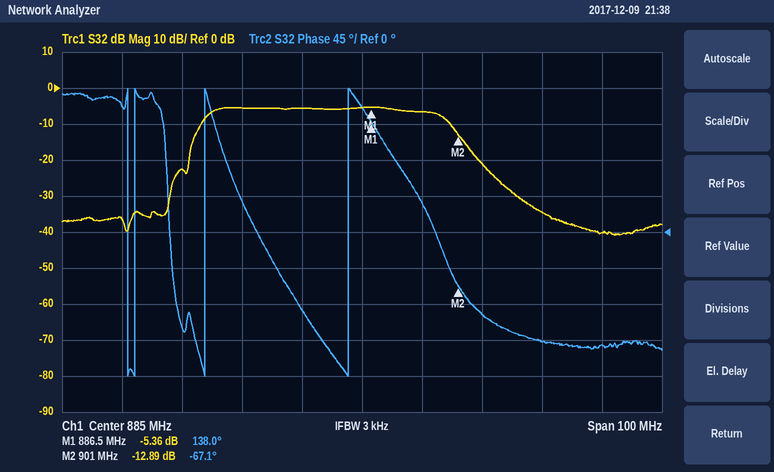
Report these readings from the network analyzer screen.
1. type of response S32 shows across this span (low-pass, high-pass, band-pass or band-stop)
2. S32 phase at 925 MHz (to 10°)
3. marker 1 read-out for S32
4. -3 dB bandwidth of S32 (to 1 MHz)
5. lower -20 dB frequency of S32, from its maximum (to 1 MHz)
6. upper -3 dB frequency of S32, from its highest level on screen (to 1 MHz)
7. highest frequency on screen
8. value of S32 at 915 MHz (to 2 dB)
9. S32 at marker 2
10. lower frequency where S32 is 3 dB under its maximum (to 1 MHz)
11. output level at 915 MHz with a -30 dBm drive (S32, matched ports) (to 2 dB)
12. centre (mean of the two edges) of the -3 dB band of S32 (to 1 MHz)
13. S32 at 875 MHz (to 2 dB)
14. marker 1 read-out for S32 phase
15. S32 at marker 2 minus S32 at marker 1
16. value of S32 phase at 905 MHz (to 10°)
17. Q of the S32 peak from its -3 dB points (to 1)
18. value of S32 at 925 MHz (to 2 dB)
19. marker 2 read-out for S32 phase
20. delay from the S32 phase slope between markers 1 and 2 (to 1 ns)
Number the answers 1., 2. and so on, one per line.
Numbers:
1. band-pass
2. -140°
3. -5.36 dB
4. 40 MHz
5. 854 MHz
6. 899 MHz
7. 935 MHz
8. -34 dB
9. -12.89 dB
10. 859 MHz
11. -64 dBm
12. 879 MHz
13. -6 dB
14. 138.0°
15. -7.53 dB
16. -100°
17. 22
18. -40 dB
19. -67.1°
20. 39 ns
